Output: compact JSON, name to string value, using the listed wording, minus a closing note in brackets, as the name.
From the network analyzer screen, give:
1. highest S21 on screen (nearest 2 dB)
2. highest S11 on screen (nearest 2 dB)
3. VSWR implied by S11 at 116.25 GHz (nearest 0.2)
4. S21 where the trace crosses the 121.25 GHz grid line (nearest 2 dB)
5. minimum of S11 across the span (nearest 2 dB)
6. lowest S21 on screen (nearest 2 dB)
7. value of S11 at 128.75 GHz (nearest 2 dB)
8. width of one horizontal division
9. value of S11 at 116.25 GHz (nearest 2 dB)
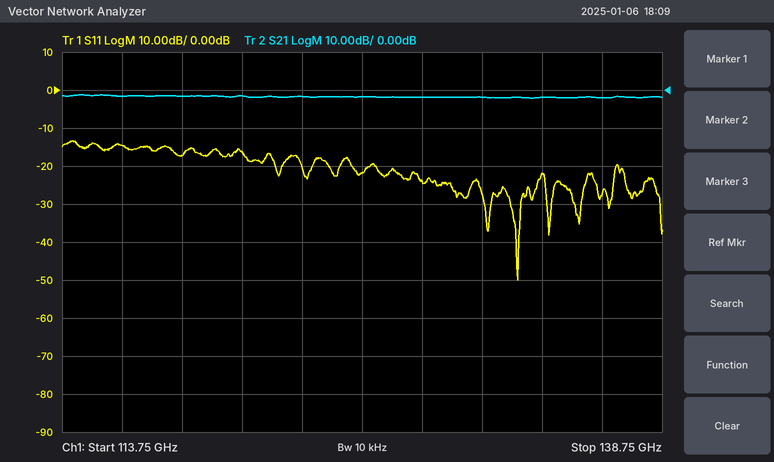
{"highest S21 on screen": "-2 dB", "highest S11 on screen": "-14 dB", "VSWR implied by S11 at 116.25 GHz": "1.4", "S21 where the trace crosses the 121.25 GHz grid line": "-2 dB", "minimum of S11 across the span": "-50 dB", "lowest S21 on screen": "-2 dB", "value of S11 at 128.75 GHz": "-24 dB", "width of one horizontal division": "2.5 GHz", "value of S11 at 116.25 GHz": "-14 dB"}
